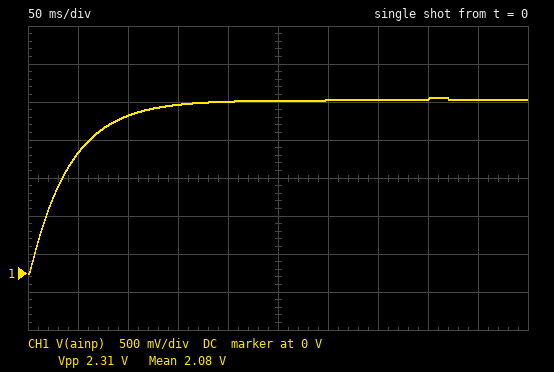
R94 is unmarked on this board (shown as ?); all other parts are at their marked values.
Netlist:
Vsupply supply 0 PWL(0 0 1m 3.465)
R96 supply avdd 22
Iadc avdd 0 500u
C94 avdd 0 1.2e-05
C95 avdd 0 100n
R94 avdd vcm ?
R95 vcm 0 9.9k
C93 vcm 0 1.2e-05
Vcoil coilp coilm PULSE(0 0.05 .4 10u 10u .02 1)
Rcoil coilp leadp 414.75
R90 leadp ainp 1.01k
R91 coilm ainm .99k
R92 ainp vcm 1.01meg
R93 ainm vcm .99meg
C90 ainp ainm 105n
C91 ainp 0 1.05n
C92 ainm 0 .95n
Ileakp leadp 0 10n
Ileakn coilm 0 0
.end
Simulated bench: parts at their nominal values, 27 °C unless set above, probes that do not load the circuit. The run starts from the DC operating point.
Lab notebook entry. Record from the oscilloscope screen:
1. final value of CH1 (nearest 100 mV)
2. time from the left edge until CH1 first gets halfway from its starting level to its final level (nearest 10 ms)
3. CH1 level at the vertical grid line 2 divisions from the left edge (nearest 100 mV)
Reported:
2.3 V
30 ms
2.1 V
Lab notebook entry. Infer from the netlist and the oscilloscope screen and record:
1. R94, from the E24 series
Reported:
5.1 kΩ
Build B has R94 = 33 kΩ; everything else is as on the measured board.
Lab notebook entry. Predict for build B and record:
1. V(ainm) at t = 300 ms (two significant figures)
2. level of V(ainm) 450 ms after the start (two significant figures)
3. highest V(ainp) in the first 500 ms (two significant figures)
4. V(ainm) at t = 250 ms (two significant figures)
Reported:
760 mV
790 mV
810 mV
740 mV
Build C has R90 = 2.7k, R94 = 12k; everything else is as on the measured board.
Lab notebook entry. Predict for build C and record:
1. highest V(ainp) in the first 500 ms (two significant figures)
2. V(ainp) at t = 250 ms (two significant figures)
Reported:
1.6 V
1.5 V
